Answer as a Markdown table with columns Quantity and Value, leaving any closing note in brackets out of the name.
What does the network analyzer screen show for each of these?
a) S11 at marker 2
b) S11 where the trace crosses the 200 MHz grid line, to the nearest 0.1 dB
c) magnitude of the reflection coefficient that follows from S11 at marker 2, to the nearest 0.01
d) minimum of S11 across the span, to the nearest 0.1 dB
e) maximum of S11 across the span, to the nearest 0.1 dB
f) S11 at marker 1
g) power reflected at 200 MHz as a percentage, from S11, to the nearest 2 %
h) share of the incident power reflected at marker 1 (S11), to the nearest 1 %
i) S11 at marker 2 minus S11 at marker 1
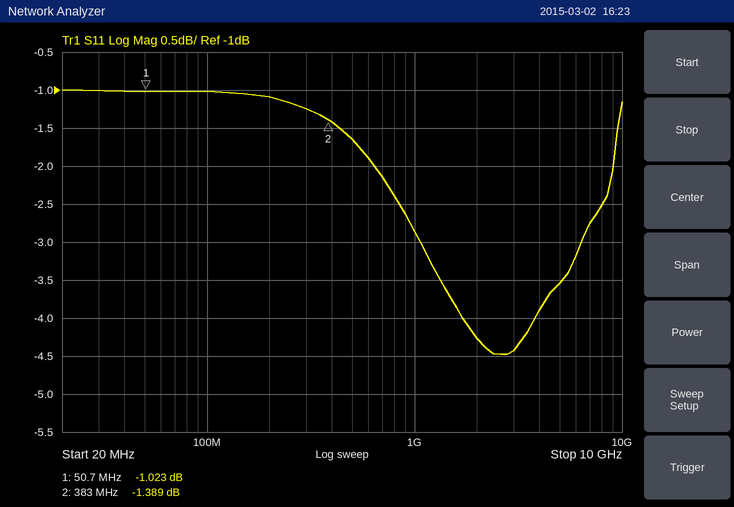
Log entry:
| Quantity | Value |
|---|---|
| S11 at marker 2 | -1.389 dB |
| S11 where the trace crosses the 200 MHz grid line, to the nearest 0.1 dB | -1.1 dB |
| magnitude of the reflection coefficient that follows from S11 at marker 2, to the nearest 0.01 | 0.85 |
| minimum of S11 across the span, to the nearest 0.1 dB | -4.5 dB |
| maximum of S11 across the span, to the nearest 0.1 dB | -1.0 dB |
| S11 at marker 1 | -1.023 dB |
| power reflected at 200 MHz as a percentage, from S11, to the nearest 2 % | 78 % |
| share of the incident power reflected at marker 1 (S11), to the nearest 1 % | 79 % |
| S11 at marker 2 minus S11 at marker 1 | -0.366 dB |
